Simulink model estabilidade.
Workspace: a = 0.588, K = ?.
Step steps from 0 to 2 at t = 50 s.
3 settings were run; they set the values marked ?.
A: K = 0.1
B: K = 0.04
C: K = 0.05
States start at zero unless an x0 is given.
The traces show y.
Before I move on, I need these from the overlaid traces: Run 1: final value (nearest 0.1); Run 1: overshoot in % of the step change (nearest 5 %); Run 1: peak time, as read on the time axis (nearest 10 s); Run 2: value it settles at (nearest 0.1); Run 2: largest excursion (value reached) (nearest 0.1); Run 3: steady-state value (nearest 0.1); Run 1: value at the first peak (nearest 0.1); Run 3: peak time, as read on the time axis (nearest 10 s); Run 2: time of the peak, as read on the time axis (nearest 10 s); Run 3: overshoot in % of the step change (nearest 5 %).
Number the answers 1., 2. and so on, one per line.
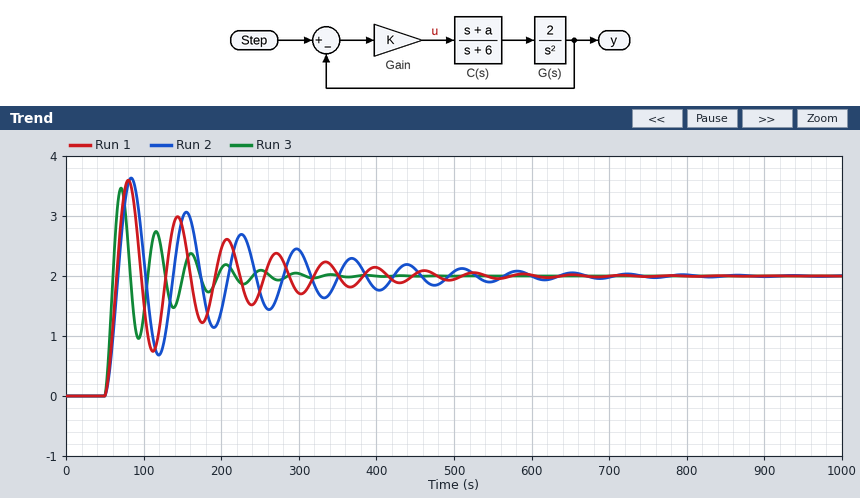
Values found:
1. 2.0
2. 80 %
3. 80 s
4. 2.0
5. 3.6
6. 2.0
7. 3.6
8. 70 s
9. 80 s
10. 75 %
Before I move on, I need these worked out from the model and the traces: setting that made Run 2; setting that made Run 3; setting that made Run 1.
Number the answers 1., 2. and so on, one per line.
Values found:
1. B
2. A
3. C
